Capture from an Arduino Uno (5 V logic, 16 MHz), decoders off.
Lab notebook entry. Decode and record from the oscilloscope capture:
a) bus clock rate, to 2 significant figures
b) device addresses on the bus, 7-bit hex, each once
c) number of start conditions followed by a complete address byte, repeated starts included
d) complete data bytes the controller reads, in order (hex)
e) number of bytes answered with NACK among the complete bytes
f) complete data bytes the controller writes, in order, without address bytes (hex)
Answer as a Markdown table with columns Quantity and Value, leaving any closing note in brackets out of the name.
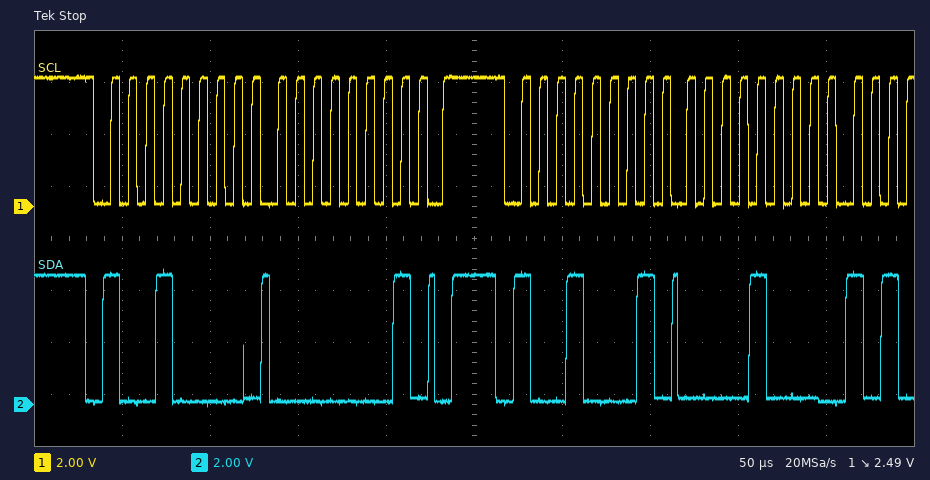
| Quantity | Value |
|---|---|
| bus clock rate, to 2 significant figures | 100 kHz |
| device addresses on the bus, 7-bit hex, each once | 0x48 |
| number of start conditions followed by a complete address byte, repeated starts included | 2 |
| complete data bytes the controller reads, in order | 08 |
| number of bytes answered with NACK among the complete bytes | 0 |
| complete data bytes the controller writes, in order, without address bytes | 01 |
